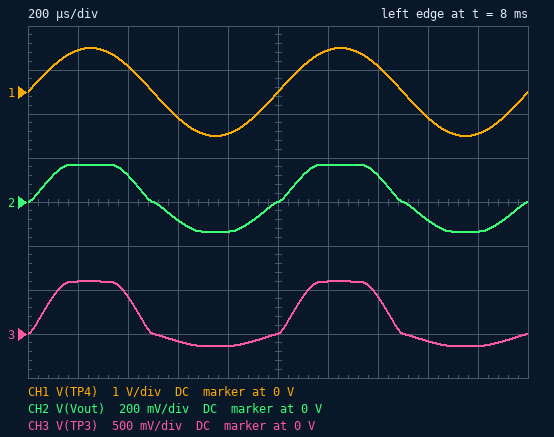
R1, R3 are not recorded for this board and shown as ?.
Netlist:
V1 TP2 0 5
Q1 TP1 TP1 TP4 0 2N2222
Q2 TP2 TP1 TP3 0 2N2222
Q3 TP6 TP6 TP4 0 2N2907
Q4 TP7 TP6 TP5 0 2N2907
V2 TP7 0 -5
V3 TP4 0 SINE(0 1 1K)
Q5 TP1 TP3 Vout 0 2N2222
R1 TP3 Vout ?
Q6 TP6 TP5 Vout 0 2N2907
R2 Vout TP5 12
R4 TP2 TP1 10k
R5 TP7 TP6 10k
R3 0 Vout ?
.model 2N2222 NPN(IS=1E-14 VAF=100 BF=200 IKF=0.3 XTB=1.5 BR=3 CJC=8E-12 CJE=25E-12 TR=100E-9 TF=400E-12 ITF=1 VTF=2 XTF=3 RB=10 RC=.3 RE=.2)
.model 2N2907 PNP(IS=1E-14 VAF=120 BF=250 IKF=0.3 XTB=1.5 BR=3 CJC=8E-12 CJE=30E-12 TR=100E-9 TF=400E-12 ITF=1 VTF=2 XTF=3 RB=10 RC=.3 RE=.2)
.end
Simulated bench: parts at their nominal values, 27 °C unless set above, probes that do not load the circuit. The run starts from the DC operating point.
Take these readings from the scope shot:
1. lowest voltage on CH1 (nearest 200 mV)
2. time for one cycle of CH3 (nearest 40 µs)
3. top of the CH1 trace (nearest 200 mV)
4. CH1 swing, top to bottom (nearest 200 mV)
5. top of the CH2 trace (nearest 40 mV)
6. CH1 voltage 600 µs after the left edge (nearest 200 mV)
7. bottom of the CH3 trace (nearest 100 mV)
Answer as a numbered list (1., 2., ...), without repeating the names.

1. -1.0 V
2. 1.00 ms
3. 1.0 V
4. 2.0 V
5. 160 mV
6. -600 mV
7. -100 mV
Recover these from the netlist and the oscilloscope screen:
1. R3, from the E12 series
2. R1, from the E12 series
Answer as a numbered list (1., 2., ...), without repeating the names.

1. 2.7 Ω
2. 6.8 Ω
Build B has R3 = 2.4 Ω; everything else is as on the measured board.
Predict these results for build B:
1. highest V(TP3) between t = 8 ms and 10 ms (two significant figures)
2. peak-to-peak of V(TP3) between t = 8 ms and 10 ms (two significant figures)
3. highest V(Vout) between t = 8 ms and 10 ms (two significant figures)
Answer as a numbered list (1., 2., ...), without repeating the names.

1. 580 mV
2. 700 mV
3. 150 mV
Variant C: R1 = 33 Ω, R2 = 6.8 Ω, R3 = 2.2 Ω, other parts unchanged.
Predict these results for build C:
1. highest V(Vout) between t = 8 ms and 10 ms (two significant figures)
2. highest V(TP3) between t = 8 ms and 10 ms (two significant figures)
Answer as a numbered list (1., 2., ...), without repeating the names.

1. 42 mV
2. 660 mV
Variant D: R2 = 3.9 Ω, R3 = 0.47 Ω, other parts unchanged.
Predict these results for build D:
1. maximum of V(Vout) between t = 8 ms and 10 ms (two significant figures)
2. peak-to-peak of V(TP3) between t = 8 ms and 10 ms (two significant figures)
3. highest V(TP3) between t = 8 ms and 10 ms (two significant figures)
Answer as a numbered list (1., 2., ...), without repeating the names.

1. 30 mV
2. 510 mV
3. 470 mV
